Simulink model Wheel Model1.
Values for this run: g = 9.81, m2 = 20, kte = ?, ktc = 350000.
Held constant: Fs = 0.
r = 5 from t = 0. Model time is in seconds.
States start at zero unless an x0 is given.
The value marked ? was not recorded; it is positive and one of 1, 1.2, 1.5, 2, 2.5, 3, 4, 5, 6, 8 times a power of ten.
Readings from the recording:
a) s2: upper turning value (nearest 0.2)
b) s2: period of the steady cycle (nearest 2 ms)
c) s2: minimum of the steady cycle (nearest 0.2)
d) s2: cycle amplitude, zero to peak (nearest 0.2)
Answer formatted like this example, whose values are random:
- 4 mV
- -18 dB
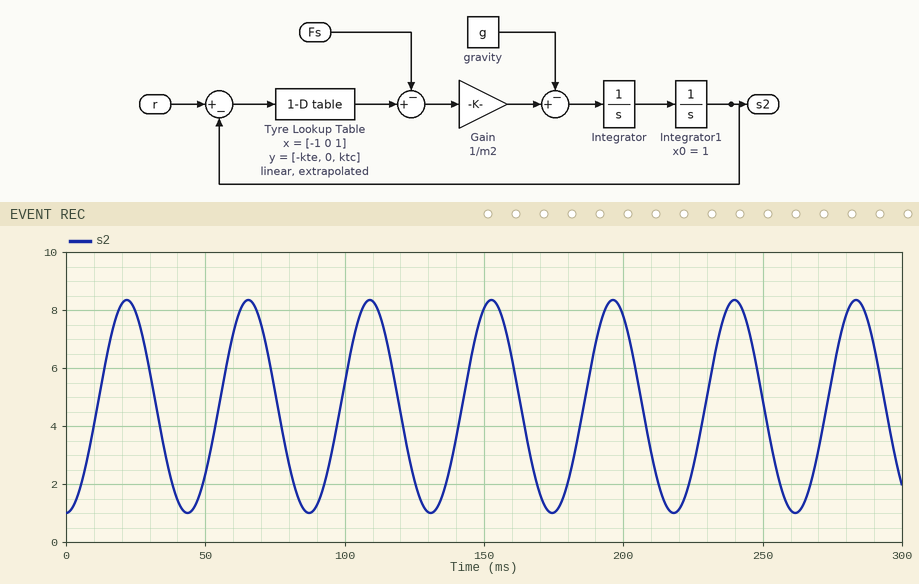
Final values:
- 8.4
- 44 ms
- 1.0
- 3.6
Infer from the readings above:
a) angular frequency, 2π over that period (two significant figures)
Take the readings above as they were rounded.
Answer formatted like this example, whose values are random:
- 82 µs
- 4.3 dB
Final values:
- 0.14 rad/ms
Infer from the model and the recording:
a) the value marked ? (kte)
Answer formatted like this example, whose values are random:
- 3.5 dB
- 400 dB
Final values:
- 500000
